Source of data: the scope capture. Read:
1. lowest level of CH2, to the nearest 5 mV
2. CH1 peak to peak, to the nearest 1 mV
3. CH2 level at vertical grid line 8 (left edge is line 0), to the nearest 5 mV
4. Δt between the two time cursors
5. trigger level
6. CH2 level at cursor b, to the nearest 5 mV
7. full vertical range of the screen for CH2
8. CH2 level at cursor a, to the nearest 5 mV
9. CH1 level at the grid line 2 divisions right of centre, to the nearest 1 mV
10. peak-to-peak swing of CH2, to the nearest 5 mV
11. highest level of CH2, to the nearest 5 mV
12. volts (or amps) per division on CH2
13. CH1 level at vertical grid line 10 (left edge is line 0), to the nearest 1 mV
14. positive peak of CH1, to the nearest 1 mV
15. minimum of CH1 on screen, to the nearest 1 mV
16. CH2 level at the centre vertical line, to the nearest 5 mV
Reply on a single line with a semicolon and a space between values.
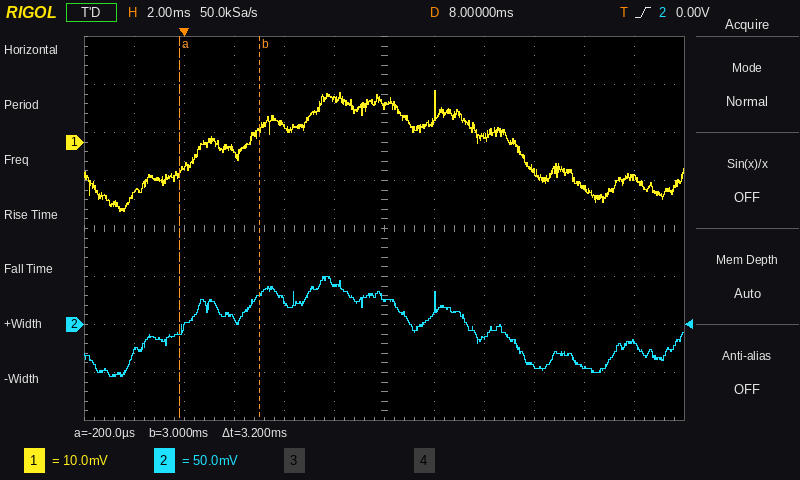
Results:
-55 mV; 25 mV; -15 mV; 3.2 ms; 0.00 V; 30 mV; 400 mV; -5 mV; 1 mV; 105 mV; 50 mV; 50 mV; -10 mV; 11 mV; -14 mV; 30 mV
